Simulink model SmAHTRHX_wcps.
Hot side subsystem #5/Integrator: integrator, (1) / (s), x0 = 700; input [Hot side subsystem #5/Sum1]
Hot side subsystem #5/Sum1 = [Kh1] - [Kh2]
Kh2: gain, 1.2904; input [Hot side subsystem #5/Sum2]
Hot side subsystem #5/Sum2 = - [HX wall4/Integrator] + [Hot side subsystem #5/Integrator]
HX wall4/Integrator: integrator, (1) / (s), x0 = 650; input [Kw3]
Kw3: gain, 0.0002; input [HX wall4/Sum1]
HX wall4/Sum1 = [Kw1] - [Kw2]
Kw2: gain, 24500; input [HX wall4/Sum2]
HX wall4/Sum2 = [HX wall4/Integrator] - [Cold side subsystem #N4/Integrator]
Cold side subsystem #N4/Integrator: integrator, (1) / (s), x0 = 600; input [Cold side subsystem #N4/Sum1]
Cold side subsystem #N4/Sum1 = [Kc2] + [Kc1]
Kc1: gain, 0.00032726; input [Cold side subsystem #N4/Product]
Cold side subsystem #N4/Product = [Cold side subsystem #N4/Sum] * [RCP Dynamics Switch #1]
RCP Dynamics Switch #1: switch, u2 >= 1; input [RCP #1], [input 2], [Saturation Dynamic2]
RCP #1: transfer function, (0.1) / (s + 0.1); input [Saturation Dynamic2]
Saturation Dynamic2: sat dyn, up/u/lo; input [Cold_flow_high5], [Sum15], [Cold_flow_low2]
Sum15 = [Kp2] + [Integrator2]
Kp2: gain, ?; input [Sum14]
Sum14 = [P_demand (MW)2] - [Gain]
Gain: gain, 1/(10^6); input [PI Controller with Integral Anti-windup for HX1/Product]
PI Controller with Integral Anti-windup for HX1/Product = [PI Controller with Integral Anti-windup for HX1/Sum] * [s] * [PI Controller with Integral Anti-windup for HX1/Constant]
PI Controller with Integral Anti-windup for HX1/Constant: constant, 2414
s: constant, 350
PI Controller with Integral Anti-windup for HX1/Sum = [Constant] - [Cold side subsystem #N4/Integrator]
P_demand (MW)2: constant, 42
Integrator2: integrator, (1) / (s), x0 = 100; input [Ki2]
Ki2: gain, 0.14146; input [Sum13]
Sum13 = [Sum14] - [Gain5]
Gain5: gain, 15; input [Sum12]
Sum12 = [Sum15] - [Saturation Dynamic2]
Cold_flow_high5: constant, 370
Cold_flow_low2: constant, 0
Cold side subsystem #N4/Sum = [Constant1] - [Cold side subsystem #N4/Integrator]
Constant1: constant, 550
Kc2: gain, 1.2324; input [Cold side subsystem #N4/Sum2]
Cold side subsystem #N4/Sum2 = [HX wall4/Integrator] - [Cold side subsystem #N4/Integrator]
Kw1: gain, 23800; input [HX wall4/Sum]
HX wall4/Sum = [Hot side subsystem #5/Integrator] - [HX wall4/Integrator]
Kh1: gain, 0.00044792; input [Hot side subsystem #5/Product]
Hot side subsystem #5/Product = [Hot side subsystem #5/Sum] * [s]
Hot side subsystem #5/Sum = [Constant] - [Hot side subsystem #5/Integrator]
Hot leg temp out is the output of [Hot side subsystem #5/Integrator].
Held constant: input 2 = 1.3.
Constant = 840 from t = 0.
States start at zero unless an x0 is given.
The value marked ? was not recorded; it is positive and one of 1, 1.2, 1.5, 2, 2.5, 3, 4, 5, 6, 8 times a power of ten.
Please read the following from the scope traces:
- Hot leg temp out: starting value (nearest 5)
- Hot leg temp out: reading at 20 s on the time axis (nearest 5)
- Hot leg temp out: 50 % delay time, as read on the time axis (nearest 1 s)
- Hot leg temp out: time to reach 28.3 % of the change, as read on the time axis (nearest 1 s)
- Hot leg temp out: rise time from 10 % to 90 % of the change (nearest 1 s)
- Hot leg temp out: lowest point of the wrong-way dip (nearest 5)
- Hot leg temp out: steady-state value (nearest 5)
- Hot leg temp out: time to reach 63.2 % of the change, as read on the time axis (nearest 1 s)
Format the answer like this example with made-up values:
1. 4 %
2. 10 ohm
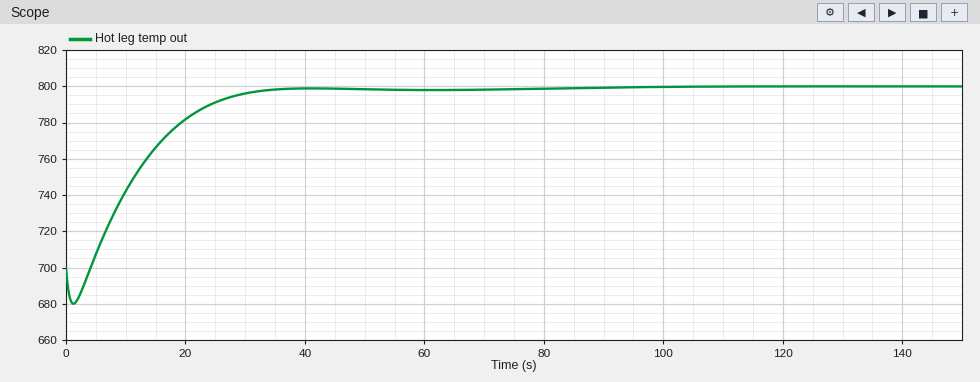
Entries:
1. 700
2. 780
3. 11 s
4. 8 s
5. 19 s
6. 680
7. 800
8. 14 s
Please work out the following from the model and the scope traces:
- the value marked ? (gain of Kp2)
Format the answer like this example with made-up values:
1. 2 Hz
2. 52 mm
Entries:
1. 2
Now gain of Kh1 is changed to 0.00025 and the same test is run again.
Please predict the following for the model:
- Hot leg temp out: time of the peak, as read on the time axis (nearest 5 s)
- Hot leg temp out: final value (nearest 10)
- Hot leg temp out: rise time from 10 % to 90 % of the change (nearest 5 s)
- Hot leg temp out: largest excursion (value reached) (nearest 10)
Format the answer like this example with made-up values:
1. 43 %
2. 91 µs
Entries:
1. 55 s
2. 800
3. 25 s
4. 800
